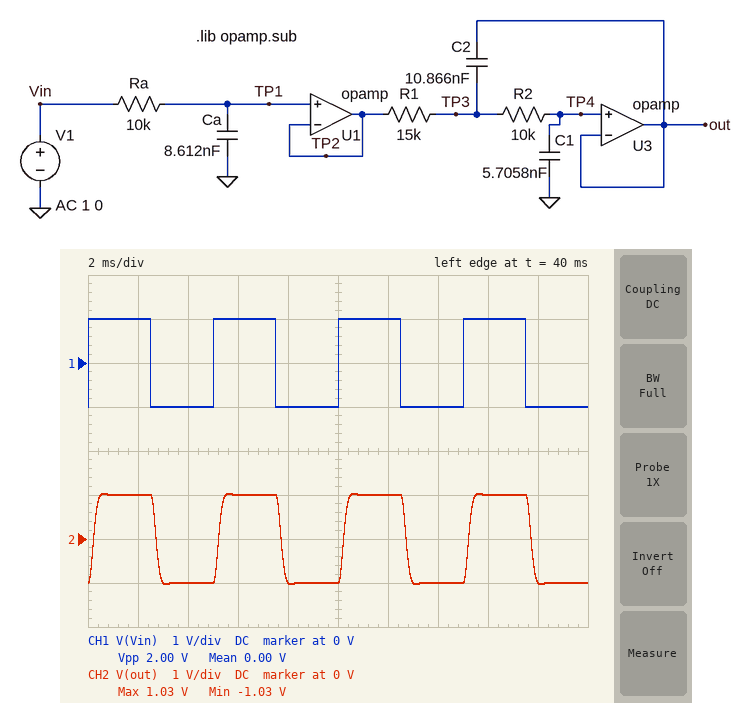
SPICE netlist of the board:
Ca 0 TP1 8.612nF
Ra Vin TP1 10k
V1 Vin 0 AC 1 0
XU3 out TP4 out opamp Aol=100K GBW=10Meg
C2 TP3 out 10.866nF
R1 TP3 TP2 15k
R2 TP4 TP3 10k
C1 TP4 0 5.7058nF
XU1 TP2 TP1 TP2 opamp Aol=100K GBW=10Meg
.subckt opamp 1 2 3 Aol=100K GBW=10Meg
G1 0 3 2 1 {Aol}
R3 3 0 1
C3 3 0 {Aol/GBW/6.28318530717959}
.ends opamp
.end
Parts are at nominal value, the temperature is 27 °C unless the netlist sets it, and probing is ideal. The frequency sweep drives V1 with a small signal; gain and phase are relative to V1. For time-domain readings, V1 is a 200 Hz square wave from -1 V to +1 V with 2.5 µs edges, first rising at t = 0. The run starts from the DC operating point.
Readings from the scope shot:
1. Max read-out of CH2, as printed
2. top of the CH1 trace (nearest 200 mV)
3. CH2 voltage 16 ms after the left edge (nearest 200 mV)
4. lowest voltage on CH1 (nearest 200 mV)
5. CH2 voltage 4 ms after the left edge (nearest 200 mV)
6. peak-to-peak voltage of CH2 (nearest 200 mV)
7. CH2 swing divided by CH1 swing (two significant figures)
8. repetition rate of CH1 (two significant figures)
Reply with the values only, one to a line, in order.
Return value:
1.03 V
1.0 V
1.0 V
-1.0 V
-1.0 V
2.0 V
1.0
200 Hz
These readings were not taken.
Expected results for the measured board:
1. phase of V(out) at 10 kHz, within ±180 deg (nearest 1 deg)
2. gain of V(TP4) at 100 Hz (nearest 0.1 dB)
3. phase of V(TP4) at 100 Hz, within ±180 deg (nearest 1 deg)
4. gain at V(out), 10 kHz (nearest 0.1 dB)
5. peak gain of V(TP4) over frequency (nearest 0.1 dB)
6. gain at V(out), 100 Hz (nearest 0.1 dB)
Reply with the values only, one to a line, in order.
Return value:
114 deg
0 dB
-8 deg
-46.1 dB
0 dB
0 dB
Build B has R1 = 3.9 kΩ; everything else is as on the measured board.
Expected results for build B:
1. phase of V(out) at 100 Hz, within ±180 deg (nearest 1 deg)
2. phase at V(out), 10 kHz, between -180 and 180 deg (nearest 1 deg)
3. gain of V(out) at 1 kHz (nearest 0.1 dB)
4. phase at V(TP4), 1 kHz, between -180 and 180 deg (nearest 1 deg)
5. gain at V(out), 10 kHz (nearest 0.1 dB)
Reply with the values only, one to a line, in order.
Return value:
-6 deg
131 deg
-1.4 dB
-57 deg
-34.7 dB
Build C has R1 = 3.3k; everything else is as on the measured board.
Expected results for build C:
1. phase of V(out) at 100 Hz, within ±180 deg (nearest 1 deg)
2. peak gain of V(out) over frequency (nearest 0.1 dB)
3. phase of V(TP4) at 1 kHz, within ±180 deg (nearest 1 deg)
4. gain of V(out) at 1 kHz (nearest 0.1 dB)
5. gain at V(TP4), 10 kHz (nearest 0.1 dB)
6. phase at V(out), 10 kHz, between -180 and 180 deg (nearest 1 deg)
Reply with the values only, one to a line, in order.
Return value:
-6 deg
0 dB
-56 deg
-1.4 dB
-33.4 dB
134 deg
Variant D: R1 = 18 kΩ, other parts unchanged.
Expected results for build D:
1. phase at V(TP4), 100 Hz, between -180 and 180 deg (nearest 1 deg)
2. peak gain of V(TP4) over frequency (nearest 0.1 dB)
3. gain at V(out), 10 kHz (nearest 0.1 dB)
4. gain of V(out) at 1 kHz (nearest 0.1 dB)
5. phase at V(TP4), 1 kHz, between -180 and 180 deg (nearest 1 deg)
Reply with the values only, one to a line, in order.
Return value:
-9 deg
0 dB
-47.7 dB
-2.3 dB
-89 deg
